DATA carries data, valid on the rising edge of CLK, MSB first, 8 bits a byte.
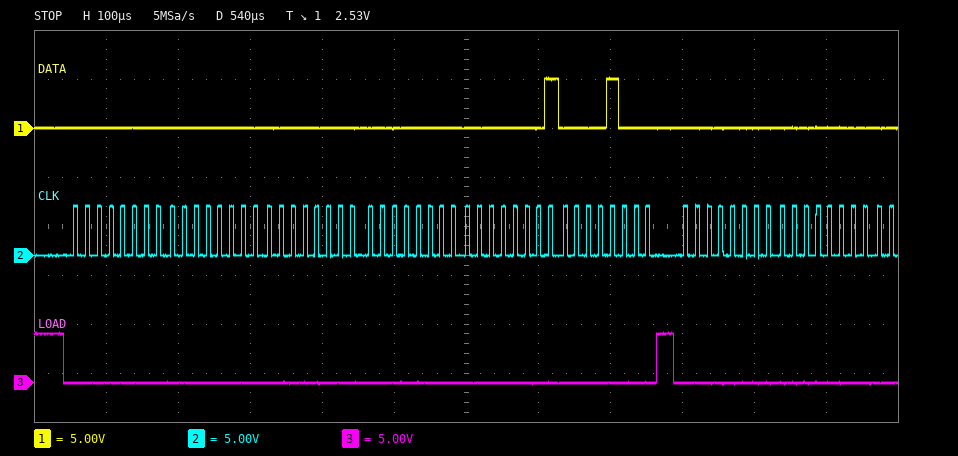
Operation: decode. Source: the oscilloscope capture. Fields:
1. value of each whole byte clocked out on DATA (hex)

00 00 00 00 01 08 00 00
